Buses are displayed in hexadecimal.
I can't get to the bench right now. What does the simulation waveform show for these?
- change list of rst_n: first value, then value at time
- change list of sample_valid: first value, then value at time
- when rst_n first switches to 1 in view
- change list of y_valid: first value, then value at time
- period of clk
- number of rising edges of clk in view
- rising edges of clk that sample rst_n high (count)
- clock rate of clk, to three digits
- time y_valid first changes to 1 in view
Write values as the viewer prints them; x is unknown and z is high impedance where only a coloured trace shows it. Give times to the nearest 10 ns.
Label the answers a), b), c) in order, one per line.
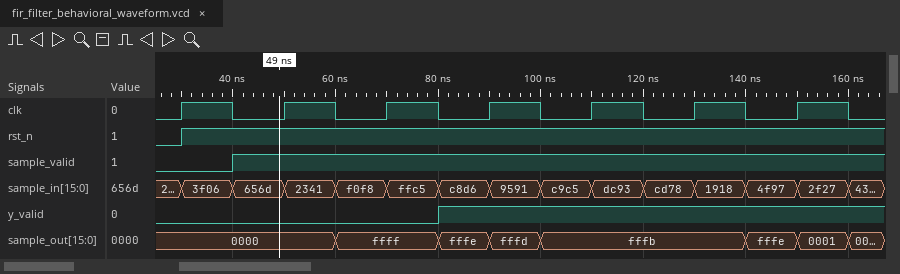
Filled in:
a) 0, 1 at 30 ns
b) 0, 1 at 40 ns
c) 30 ns
d) 0, 1 at 80 ns
e) 20 ns
f) 7
g) 6
h) 50.0 MHz
i) 80 ns
